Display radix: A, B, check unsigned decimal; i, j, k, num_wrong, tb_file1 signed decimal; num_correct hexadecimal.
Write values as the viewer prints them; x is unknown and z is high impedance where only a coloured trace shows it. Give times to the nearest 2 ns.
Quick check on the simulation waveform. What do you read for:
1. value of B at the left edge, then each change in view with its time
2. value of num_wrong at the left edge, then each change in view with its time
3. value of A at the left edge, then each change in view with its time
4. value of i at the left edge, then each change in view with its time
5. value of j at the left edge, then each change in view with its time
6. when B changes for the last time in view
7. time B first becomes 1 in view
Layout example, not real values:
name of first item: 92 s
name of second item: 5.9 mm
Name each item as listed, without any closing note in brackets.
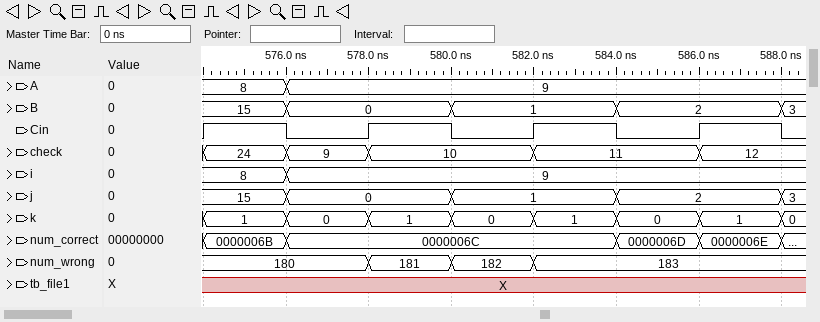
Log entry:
value of B at the left edge, then each change in view with its time: 15, 0 at 576 ns, 1 at 580 ns, 2 at 584 ns, 3 at 588 ns
value of num_wrong at the left edge, then each change in view with its time: 180, 181 at 578 ns, 182 at 580 ns, 183 at 582 ns
value of A at the left edge, then each change in view with its time: 8, 9 at 576 ns
value of i at the left edge, then each change in view with its time: 8, 9 at 576 ns
value of j at the left edge, then each change in view with its time: 15, 0 at 576 ns, 1 at 580 ns, 2 at 584 ns, 3 at 588 ns
when B changes for the last time in view: 588 ns
time B first becomes 1 in view: 580 ns
